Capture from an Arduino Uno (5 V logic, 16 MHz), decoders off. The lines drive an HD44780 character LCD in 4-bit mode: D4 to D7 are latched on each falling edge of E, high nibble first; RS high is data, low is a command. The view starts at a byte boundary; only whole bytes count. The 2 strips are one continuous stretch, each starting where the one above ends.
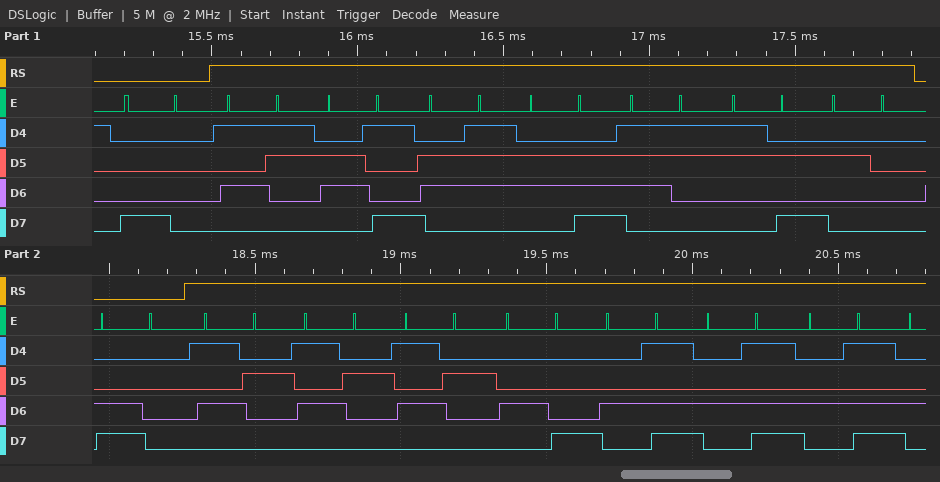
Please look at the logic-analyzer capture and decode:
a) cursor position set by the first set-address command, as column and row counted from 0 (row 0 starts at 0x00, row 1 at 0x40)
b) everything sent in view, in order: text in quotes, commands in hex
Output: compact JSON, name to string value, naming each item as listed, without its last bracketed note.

{"cursor position set by the first set-address command, as column and row counted from 0": "column 0, row 0", "everything sent in view, in order: text in quotes, commands in hex": "0x80 \"Signs: \" 0xC0 \"RRRHMMM\""}
